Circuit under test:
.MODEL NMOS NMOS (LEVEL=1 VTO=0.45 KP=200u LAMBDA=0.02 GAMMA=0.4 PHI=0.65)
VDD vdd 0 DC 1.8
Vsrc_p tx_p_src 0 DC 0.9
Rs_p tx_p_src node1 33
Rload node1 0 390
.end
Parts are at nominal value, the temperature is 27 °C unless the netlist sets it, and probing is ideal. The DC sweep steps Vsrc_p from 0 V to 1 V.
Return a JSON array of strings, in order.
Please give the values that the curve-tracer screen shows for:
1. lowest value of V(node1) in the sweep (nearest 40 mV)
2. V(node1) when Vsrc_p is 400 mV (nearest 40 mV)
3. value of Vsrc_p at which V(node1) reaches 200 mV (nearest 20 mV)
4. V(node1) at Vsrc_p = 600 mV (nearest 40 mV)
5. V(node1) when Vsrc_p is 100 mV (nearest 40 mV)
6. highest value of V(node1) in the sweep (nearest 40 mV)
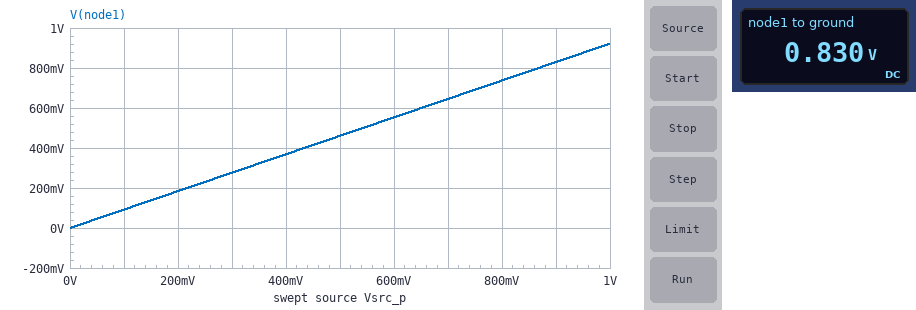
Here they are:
["0 V", "360 mV", "220 mV", "560 mV", "80 mV", "920 mV"]
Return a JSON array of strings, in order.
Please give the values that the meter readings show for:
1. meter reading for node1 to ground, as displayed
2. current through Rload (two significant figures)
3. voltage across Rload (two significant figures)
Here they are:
["0.830 V", "2.1 mA", "830 mV"]
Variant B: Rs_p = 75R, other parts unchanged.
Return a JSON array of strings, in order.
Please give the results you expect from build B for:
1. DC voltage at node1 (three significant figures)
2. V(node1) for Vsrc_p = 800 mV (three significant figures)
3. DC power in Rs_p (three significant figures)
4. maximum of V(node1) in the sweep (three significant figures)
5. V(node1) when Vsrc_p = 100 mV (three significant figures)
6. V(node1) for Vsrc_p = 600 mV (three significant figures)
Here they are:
["755 mV", "671 mV", "281 µW", "839 mV", "83.9 mV", "503 mV"]
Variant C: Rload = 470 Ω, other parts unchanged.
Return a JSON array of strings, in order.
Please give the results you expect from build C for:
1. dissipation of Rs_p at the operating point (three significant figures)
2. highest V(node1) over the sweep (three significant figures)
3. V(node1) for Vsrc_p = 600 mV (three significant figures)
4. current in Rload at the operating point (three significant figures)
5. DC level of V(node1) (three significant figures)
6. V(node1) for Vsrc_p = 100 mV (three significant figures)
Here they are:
["106 µW", "934 mV", "561 mV", "1.79 mA", "841 mV", "93.4 mV"]
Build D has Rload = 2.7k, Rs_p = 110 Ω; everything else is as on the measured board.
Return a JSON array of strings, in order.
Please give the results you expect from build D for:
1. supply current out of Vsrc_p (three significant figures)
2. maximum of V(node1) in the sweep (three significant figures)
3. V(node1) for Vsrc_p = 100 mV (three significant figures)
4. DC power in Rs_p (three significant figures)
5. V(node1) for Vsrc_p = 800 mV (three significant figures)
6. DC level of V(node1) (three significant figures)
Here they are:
["320 µA", "961 mV", "96.1 mV", "11.3 µW", "769 mV", "865 mV"]
